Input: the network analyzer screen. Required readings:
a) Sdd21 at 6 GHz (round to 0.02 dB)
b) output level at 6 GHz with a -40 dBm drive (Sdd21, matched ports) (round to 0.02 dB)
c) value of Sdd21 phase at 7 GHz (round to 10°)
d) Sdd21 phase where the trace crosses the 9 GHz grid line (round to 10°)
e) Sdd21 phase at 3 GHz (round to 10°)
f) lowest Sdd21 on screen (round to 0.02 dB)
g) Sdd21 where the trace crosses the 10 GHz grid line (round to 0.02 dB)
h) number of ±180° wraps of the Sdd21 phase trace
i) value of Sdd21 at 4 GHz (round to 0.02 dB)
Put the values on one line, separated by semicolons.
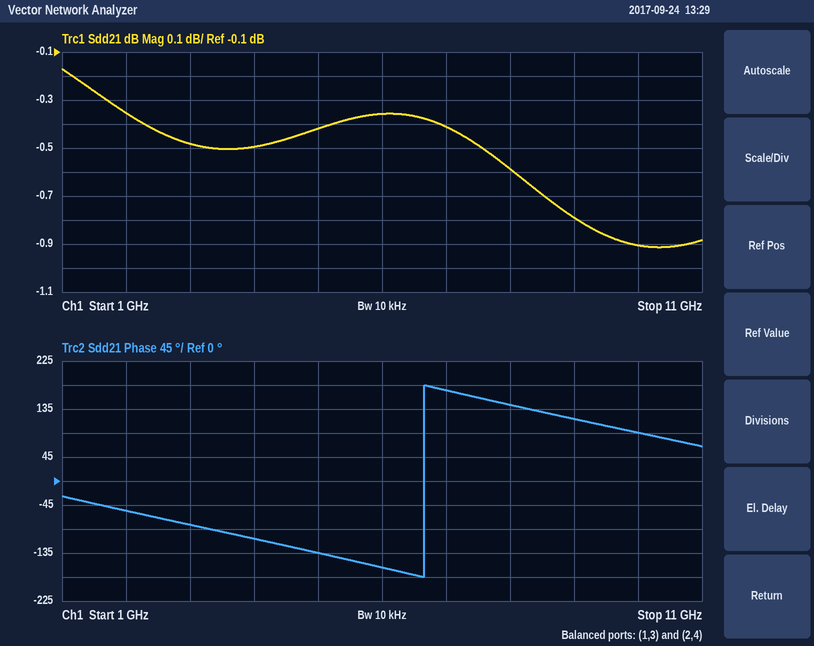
-0.36 dB; -40.36 dBm; 170°; 120°; -80°; -0.92 dB; -0.90 dB; 1; -0.50 dB
